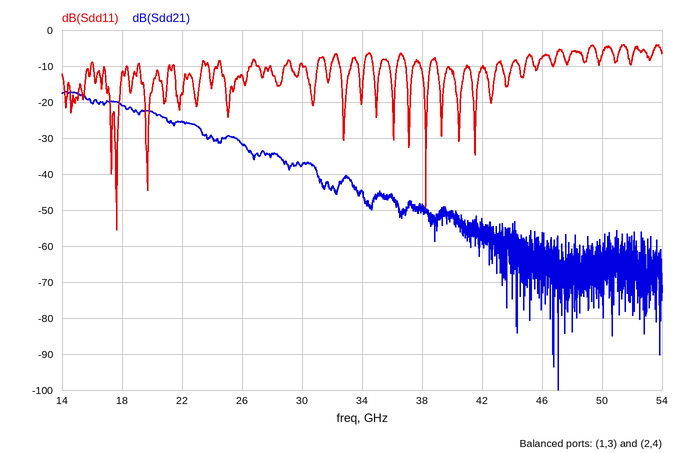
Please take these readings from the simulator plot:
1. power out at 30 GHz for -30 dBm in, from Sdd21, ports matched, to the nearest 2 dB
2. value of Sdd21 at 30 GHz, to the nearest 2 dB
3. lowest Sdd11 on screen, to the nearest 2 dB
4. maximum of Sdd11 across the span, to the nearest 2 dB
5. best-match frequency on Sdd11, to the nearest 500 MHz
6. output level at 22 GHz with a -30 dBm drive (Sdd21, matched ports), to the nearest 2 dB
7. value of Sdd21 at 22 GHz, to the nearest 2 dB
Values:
-68 dBm
-38 dB
-56 dB
-4 dB
17.5 GHz
-56 dBm
-26 dB
